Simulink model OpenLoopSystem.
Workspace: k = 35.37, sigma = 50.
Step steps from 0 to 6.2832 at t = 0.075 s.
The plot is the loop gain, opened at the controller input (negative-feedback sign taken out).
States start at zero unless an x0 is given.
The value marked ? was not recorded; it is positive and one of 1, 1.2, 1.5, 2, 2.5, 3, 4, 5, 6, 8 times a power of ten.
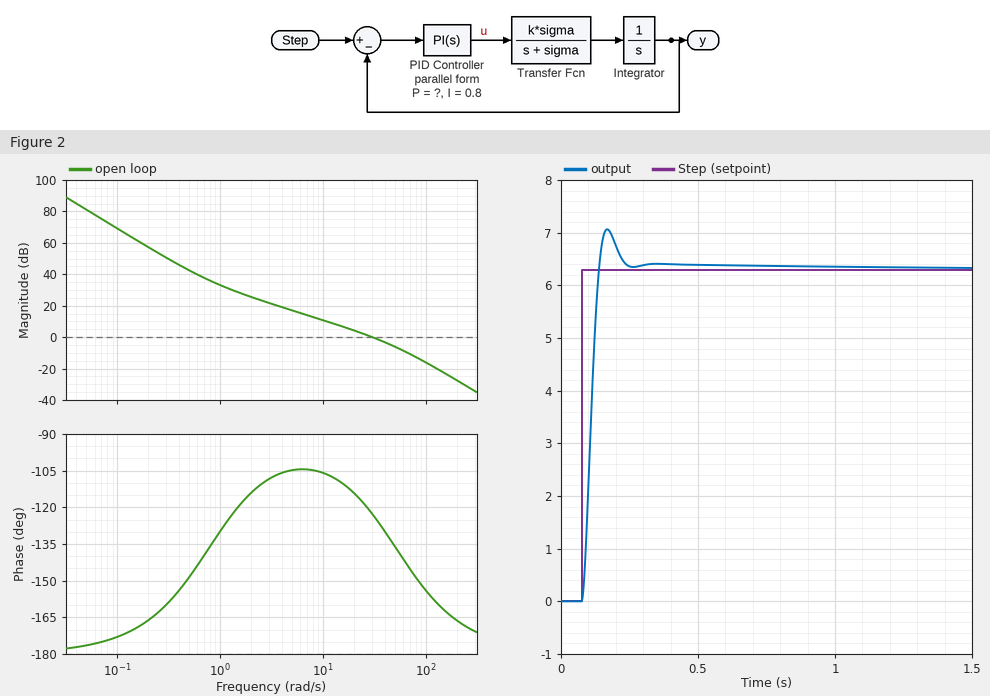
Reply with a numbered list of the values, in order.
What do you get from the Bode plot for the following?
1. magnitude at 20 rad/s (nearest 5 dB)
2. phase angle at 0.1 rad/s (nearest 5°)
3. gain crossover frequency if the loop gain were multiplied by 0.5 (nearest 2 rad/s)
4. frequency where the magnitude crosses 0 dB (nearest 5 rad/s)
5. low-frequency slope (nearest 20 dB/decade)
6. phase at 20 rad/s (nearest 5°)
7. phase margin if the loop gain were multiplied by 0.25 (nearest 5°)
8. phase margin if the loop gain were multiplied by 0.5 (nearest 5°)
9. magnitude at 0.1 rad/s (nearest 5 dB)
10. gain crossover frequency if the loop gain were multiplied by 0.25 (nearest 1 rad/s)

1. 5 dB
2. -175°
3. 16 rad/s
4. 30 rad/s
5. -40 dB/decade
6. -115°
7. 75°
8. 70°
9. 70 dB
10. 9 rad/s
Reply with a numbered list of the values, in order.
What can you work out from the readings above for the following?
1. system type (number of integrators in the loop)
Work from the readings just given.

1. 2
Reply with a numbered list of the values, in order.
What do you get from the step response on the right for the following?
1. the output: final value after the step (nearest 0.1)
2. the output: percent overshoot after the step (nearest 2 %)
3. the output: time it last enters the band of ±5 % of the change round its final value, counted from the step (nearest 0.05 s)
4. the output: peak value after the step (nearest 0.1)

1. 6.3
2. 12 %
3. 0.15 s
4. 7.1
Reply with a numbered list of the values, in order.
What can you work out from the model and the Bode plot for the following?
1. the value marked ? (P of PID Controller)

1. 1
